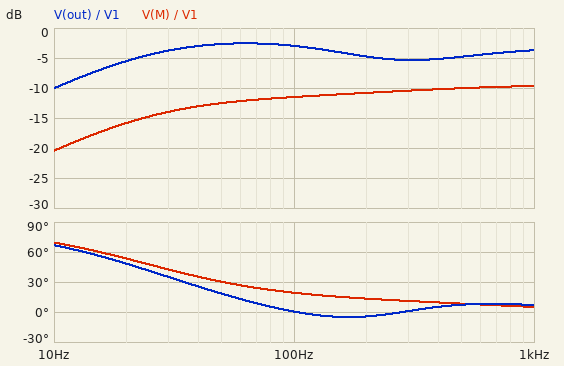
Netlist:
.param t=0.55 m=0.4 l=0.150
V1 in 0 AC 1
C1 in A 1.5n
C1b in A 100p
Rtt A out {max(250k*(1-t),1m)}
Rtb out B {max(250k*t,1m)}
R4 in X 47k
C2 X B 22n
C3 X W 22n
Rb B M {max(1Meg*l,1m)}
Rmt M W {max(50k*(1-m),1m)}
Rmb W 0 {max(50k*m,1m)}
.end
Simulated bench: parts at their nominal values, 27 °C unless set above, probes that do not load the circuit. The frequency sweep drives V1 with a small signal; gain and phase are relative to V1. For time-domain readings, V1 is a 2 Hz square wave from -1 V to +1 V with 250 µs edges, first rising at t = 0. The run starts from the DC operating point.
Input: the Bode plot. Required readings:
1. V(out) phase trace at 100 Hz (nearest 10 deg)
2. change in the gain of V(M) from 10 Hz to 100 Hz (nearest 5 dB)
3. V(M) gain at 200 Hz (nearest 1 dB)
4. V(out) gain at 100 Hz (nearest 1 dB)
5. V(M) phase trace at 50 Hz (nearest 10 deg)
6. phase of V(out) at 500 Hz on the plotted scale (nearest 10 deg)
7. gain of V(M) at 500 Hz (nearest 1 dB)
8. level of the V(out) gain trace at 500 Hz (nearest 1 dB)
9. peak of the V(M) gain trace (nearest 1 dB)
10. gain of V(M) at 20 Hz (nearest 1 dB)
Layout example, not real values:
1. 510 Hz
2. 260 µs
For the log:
1. 0 deg
2. 10 dB
3. -11 dB
4. -3 dB
5. 30 deg
6. 10 deg
7. -10 dB
8. -5 dB
9. -10 dB
10. -16 dB
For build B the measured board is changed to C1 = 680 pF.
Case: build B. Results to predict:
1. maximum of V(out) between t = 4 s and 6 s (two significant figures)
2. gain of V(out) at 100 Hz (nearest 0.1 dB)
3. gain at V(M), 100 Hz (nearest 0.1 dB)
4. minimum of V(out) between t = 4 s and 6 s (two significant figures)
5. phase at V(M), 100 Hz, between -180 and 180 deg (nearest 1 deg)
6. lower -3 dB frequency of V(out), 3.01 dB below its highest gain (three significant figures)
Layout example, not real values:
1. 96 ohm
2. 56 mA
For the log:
1. 1.2 V
2. -3.2 dB
3. -11.6 dB
4. -1.2 V
5. 19 deg
6. 20.4 Hz
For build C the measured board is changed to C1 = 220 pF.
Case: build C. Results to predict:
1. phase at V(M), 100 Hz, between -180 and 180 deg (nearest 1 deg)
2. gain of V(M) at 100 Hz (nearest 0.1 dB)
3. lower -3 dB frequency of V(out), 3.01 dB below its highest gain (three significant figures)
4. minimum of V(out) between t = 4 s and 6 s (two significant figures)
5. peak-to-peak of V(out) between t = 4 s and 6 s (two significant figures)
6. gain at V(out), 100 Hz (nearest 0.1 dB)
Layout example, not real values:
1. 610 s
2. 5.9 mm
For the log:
1. 19 deg
2. -11.6 dB
3. 20.8 Hz
4. -1.2 V
5. 2.3 V
6. -3.2 dB
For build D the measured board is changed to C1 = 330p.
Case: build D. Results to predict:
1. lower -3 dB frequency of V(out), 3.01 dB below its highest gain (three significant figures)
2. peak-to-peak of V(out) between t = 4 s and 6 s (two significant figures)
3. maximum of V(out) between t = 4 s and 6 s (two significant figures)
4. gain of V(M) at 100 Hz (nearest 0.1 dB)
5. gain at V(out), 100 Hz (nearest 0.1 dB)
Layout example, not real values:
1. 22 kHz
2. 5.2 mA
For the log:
1. 20.7 Hz
2. 2.3 V
3. 1.2 V
4. -11.6 dB
5. -3.2 dB
